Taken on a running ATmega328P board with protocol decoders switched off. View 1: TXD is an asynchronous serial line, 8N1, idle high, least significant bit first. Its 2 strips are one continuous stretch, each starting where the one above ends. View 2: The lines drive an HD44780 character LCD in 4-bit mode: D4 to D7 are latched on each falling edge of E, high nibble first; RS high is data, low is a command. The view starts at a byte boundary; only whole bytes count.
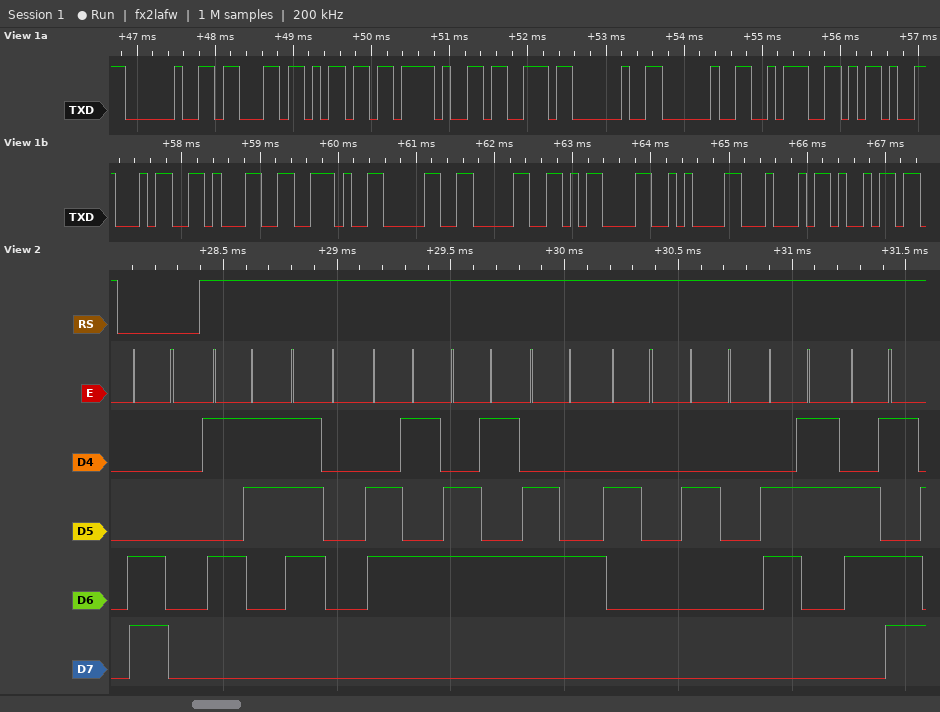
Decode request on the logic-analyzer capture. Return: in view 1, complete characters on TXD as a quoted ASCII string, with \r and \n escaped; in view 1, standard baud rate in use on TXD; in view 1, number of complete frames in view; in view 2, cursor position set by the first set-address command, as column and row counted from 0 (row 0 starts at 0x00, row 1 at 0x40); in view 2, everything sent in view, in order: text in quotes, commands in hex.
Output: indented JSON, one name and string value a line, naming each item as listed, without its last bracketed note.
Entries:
{
  "in view 1, complete characters on TXD as a quoted ASCII string, with \\r and \\n escaped": "\" cm/s  :-41.00\\r\\nDi\"",
  "in view 1, standard baud rate in use on TXD": "9600 baud",
  "in view 1, number of complete frames in view": "18",
  "in view 2, cursor position set by the first set-address command, as column and row counted from 0": "column 0, row 1",
  "in view 2, everything sent in view, in order: text in quotes, commands in hex": "0xC0 \"Speed  cm\""
}
